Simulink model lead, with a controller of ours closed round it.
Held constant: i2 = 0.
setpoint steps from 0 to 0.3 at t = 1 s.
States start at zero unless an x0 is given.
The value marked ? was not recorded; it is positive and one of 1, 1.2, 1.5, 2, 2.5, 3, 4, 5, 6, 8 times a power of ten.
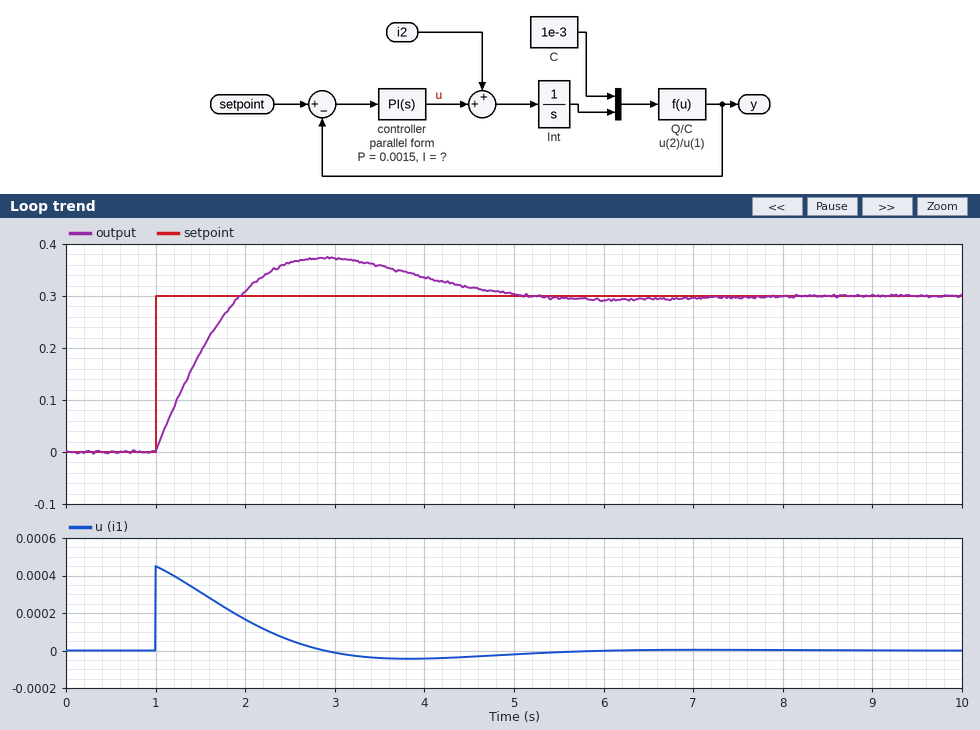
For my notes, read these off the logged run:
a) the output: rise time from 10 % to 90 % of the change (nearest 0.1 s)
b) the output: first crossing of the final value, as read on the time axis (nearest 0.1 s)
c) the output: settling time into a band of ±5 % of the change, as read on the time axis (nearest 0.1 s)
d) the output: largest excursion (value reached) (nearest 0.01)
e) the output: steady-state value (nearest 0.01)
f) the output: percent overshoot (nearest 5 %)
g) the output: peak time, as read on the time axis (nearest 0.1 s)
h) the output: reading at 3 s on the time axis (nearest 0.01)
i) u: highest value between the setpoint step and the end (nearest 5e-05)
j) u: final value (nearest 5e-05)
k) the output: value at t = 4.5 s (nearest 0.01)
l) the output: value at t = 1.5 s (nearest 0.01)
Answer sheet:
0.7 s
1.9 s
4.6 s
0.37
0.30
25 %
2.9 s
0.37
0.00045
0.00000
0.32
0.19
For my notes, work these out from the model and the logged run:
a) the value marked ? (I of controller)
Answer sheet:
0.0015
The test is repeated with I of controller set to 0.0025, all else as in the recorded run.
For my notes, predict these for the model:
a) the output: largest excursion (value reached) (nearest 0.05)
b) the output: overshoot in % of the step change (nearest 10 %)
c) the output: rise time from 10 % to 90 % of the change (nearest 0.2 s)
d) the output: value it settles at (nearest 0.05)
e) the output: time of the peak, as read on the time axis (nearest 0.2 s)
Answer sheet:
0.40
30 %
0.6 s
0.30
2.6 s
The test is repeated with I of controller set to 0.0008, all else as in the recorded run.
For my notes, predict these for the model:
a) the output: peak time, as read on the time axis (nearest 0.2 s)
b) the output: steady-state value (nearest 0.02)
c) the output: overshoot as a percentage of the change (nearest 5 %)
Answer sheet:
3.4 s
0.30
15 %
